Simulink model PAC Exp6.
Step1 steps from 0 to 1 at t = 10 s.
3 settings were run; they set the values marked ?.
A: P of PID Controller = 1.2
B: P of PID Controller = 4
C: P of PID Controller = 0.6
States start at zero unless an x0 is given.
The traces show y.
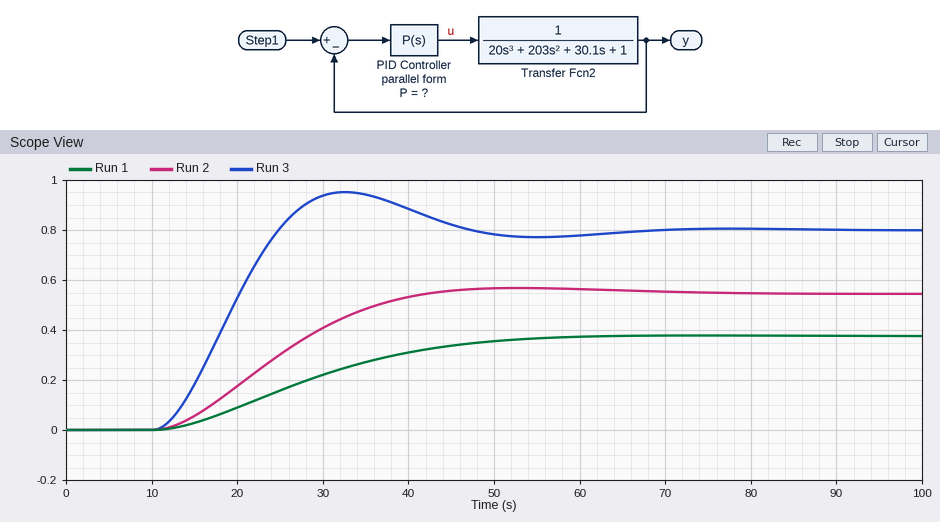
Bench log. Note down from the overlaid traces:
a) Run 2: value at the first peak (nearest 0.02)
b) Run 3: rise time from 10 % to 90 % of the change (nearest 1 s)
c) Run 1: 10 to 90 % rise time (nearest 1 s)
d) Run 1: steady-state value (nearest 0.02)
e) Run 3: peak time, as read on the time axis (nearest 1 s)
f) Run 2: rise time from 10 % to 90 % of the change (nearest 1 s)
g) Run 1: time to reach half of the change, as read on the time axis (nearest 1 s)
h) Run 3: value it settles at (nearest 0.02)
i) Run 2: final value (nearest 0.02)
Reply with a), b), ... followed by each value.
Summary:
a) 0.56
b) 10 s
c) 29 s
d) 0.38
e) 33 s
f) 21 s
g) 27 s
h) 0.80
i) 0.54
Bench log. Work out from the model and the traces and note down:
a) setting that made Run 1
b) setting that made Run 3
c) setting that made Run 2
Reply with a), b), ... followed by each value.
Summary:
a) C
b) B
c) A
